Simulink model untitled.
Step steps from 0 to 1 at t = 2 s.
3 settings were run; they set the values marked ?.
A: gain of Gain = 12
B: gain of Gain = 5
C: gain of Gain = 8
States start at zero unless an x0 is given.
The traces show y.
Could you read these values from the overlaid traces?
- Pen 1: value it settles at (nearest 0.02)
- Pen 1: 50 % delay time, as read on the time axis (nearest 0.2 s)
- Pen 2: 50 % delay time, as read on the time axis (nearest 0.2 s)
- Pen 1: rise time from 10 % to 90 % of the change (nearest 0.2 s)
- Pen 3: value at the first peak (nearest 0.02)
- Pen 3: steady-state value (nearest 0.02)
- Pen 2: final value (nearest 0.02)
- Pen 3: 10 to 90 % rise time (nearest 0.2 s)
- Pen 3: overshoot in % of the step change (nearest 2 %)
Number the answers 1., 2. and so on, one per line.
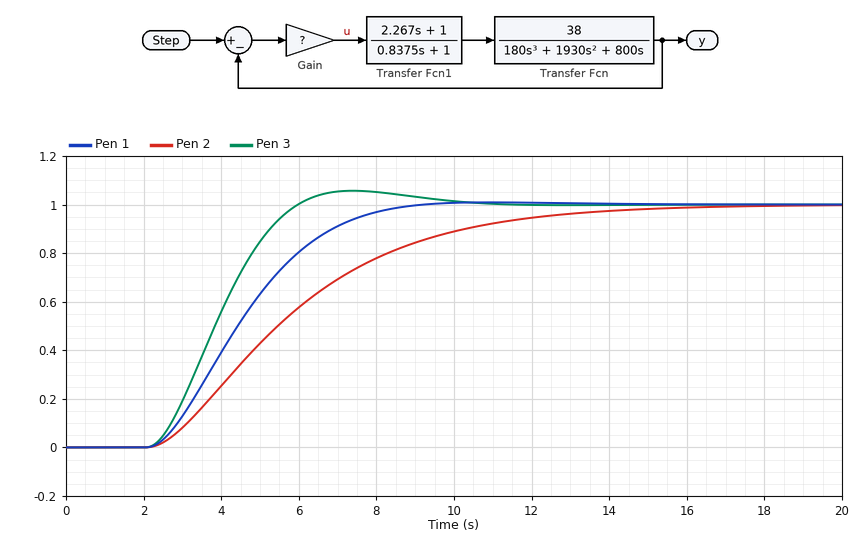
1. 1.00
2. 4.4 s
3. 5.4 s
4. 4.0 s
5. 1.06
6. 1.00
7. 1.00
8. 2.6 s
9. 6 %
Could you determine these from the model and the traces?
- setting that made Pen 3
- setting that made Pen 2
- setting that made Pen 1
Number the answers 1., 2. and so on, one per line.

1. A
2. B
3. C
